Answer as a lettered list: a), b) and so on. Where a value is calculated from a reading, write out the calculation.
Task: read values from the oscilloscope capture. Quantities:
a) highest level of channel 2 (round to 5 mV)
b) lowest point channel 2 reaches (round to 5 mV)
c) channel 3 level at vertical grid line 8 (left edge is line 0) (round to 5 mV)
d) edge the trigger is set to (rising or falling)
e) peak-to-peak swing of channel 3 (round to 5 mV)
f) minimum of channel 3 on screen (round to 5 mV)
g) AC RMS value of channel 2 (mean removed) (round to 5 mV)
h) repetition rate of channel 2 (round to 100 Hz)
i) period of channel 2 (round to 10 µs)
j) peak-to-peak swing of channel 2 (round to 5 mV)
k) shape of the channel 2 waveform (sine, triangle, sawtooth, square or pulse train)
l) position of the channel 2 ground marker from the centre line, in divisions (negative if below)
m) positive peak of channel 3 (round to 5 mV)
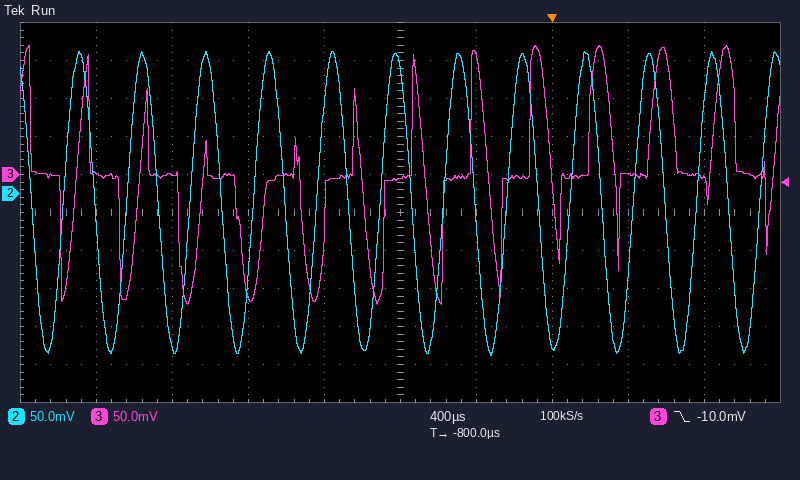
a) 185 mV
b) -215 mV
c) 0 mV
d) falling
e) 170 mV − (-170 mV) = 340 mV
f) -170 mV
g) 400 mV / (2√2) ≈ 141 mV, so 140 mV to the nearest 5 mV
h) 1 / 330 µs ≈ 3.0 kHz
i) 330 µs
j) 185 mV − (-215 mV) = 400 mV
k) sine
l) +0.5 div
m) 170 mV
